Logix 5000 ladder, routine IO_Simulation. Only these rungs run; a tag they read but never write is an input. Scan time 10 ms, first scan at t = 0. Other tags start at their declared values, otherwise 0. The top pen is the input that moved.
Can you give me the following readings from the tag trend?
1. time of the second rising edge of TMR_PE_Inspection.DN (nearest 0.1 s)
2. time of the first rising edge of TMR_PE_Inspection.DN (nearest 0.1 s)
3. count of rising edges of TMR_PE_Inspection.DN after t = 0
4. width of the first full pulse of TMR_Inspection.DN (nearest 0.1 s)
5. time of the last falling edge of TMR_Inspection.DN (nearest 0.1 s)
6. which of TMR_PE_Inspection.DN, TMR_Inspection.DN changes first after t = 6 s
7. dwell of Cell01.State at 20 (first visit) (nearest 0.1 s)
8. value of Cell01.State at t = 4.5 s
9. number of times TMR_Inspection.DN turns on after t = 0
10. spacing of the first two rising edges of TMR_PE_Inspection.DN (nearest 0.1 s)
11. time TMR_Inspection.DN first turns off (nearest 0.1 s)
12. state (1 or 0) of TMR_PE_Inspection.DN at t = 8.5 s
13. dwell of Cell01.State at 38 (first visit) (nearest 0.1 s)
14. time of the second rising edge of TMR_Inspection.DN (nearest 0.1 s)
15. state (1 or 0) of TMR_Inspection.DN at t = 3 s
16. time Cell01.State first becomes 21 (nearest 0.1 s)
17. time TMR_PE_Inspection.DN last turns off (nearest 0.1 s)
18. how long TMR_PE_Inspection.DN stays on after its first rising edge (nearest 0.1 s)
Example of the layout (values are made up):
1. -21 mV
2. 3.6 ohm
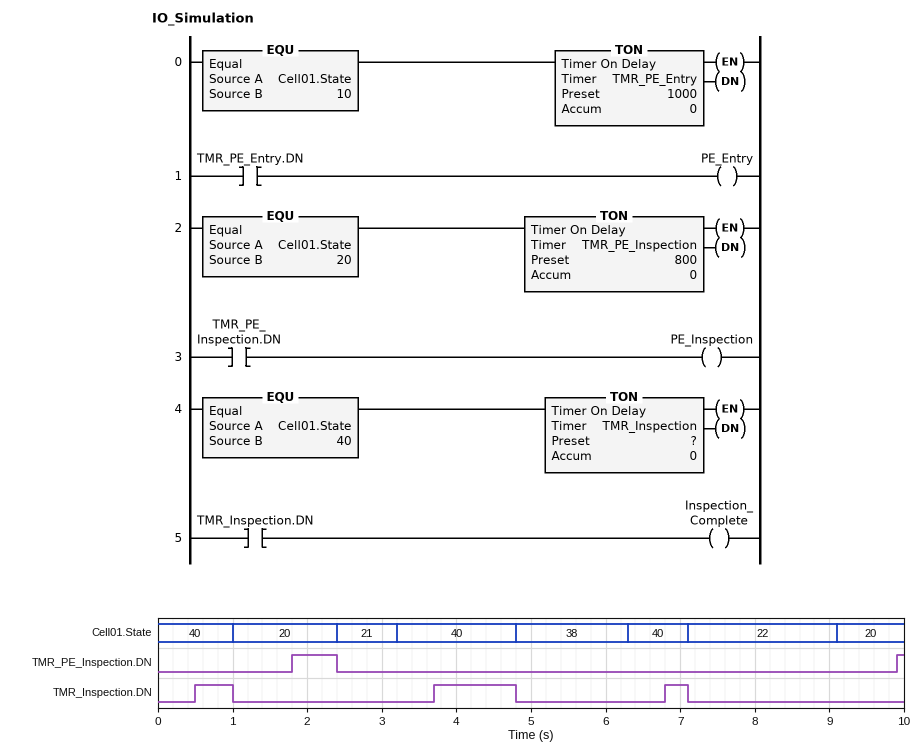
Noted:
1. 9.9 s
2. 1.8 s
3. 2
4. 0.5 s
5. 7.1 s
6. TMR_Inspection.DN
7. 1.4 s
8. 40
9. 3
10. 8.1 s
11. 1.0 s
12. 0
13. 1.5 s
14. 3.7 s
15. 0
16. 2.4 s
17. 2.4 s
18. 0.6 s
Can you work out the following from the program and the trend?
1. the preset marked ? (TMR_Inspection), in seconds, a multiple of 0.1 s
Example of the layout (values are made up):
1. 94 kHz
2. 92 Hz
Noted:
1. 0.5 s
